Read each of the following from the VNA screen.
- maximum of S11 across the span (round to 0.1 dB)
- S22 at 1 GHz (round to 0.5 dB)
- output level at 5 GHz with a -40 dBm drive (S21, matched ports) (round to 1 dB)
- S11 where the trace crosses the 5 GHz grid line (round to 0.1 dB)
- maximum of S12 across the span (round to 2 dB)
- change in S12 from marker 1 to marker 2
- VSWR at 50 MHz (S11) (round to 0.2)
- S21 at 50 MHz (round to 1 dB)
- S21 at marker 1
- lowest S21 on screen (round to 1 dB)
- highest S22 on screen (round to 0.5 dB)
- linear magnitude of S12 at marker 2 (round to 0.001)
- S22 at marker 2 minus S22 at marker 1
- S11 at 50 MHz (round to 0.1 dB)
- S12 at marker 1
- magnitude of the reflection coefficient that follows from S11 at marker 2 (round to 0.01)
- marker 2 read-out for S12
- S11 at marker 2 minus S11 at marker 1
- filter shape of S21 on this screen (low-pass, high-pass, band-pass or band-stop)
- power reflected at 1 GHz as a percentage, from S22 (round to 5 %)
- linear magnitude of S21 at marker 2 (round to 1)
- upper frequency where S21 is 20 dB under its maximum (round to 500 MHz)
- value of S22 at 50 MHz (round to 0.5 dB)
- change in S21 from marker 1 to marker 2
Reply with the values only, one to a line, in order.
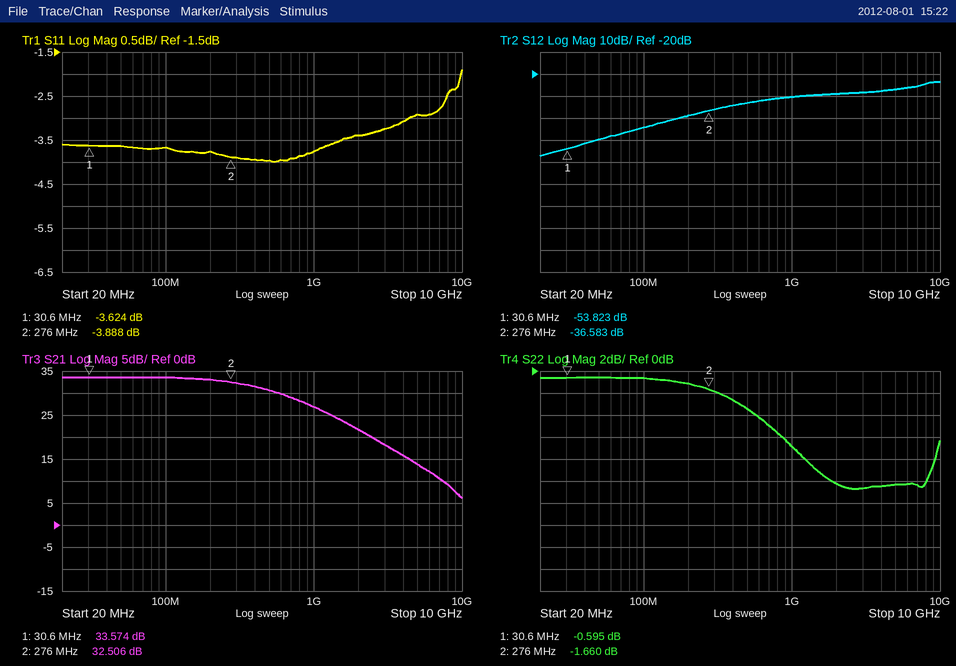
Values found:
-1.9 dB
-7.0 dB
-26 dBm
-2.9 dB
-24 dB
17.240 dB
4.8
34 dB
33.574 dB
6 dB
-0.5 dB
0.015
-1.065 dB
-3.6 dB
-53.823 dB
0.64
-36.583 dB
-0.264 dB
low-pass
20 %
42
5.0 GHz
-0.5 dB
-1.068 dB
